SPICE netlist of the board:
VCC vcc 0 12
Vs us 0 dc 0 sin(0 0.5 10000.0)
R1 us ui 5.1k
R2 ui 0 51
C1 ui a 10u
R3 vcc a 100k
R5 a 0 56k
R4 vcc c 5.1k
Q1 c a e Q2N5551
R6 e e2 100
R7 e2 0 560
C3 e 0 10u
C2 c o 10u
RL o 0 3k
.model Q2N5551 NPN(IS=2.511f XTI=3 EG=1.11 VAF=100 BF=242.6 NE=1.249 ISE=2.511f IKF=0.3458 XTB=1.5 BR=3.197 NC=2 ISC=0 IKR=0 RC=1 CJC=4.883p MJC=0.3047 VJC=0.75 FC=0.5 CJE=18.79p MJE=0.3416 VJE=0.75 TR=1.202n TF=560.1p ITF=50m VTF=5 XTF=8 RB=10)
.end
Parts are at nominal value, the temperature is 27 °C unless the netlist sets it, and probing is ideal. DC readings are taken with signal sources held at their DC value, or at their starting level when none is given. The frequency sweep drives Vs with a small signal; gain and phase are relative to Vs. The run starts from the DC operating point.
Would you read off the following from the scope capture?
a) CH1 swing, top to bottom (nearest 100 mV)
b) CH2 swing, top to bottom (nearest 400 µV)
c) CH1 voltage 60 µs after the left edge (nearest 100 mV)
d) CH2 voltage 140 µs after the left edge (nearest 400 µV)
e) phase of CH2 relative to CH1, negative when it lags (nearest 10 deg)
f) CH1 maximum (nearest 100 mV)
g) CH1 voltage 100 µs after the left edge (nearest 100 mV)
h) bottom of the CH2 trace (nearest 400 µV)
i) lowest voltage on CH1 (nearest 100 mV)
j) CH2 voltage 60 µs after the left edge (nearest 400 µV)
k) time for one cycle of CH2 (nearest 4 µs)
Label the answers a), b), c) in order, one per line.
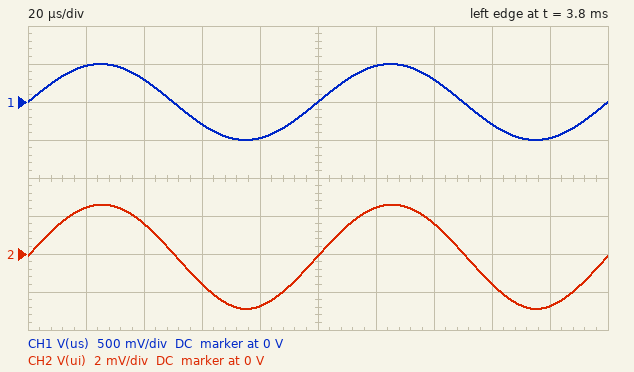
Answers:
a) 1.0 V
b) 5.6 mV
c) -300 mV
d) 1.6 mV
e) 0 deg
f) 500 mV
g) 0 V
h) -2.8 mV
i) -500 mV
j) -1.6 mV
k) 100 µs
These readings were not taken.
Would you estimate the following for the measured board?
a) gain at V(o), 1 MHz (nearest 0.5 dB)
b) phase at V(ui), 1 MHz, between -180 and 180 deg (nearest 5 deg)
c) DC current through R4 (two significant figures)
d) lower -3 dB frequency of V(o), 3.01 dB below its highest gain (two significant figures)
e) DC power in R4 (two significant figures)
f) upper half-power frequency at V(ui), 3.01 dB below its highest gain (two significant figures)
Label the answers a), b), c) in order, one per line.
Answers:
a) -26.5 dB
b) 0 deg
c) 2.1 mA
d) 350 Hz
e) 22 mW
f) 510 Hz
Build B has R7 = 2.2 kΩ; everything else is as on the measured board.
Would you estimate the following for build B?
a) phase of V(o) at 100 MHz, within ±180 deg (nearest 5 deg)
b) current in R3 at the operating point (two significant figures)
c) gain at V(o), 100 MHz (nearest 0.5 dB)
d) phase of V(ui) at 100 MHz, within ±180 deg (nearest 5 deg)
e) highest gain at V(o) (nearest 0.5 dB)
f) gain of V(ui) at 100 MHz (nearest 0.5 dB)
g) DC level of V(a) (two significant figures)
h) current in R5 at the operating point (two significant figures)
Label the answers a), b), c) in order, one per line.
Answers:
a) 65 deg
b) 81 µA
c) -27.5 dB
d) -20 deg
e) -0.5 dB
f) -50.0 dB
g) 3.9 V
h) 69 µA
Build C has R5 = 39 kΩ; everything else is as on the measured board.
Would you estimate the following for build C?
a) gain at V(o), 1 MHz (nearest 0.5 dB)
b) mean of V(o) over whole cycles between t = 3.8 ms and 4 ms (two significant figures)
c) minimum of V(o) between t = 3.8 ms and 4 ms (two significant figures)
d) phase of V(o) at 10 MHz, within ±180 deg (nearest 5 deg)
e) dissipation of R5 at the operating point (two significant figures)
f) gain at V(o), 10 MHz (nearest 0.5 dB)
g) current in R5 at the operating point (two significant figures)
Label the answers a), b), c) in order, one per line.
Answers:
a) -22.5 dB
b) 27 mV
c) -30 mV
d) 150 deg
e) 110 µW
f) -23.5 dB
g) 54 µA
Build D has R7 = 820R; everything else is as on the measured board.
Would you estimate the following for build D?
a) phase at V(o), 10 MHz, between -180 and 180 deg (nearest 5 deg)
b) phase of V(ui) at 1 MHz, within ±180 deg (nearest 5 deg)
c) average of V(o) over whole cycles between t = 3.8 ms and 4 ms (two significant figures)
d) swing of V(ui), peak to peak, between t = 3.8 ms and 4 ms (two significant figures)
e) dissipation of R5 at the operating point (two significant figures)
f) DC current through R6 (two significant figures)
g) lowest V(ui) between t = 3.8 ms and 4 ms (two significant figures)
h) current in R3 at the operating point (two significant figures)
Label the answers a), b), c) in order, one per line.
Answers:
a) 150 deg
b) 0 deg
c) 18 mV
d) 5.9 mV
e) 120 µW
f) 2.0 mA
g) -3.3 mV
h) 94 µA
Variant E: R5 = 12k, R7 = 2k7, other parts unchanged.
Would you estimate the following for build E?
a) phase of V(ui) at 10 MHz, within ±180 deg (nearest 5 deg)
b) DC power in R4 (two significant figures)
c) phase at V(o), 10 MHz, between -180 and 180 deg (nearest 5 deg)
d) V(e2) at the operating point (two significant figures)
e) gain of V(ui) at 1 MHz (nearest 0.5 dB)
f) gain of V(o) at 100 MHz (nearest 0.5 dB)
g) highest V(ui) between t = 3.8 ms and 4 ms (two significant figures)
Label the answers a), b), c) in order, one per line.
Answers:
a) -10 deg
b) 240 µW
c) 150 deg
d) 590 mV
e) -40.0 dB
f) -31.5 dB
g) 4.9 mV
